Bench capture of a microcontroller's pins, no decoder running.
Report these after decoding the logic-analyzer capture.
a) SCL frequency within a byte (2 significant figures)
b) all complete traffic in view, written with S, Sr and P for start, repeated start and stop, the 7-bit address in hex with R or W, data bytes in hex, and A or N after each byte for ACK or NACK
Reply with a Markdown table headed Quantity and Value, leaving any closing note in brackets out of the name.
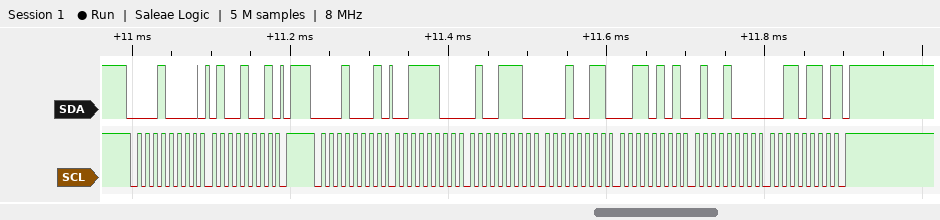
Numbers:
| Quantity | Value |
|---|---|
| SCL frequency within a byte | 100 kHz |
| all complete traffic in view, written with S, Sr and P for start, repeated start and stop, the 7-bit address in hex with R or W, data bytes in hex, and A or N after each byte for ACK or NACK | S 08W A 49 A P S 08R A 3C A 4E A 13 A 35 A 48 A 36 N P |
